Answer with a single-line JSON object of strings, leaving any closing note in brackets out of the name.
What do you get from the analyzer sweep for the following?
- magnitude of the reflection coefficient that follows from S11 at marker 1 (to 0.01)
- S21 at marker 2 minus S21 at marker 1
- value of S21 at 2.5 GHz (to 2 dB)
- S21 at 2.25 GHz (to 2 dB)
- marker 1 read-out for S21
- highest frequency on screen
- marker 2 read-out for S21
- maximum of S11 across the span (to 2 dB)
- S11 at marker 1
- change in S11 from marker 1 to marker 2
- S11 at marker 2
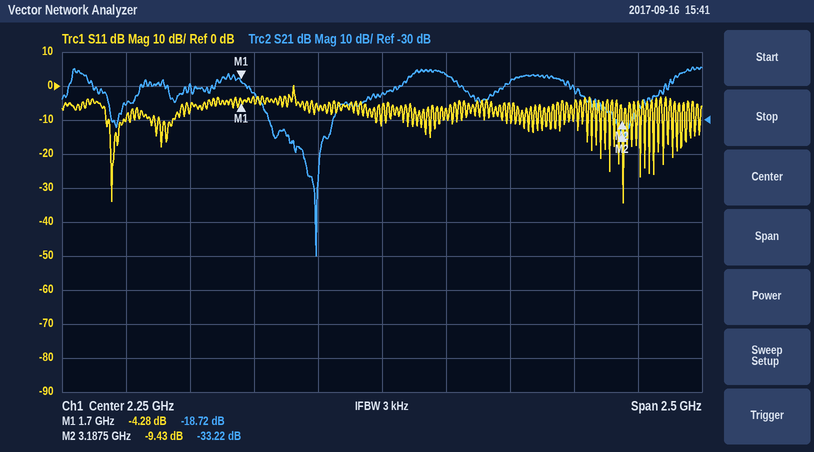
{"magnitude of the reflection coefficient that follows from S11 at marker 1": "0.61", "S21 at marker 2 minus S21 at marker 1": "-14.50 dB", "value of S21 at 2.5 GHz": "-16 dB", "S21 at 2.25 GHz": "-22 dB", "marker 1 read-out for S21": "-18.72 dB", "highest frequency on screen": "3.5 GHz", "marker 2 read-out for S21": "-33.22 dB", "maximum of S11 across the span": "0 dB", "S11 at marker 1": "-4.28 dB", "change in S11 from marker 1 to marker 2": "-5.15 dB", "S11 at marker 2": "-9.43 dB"}
